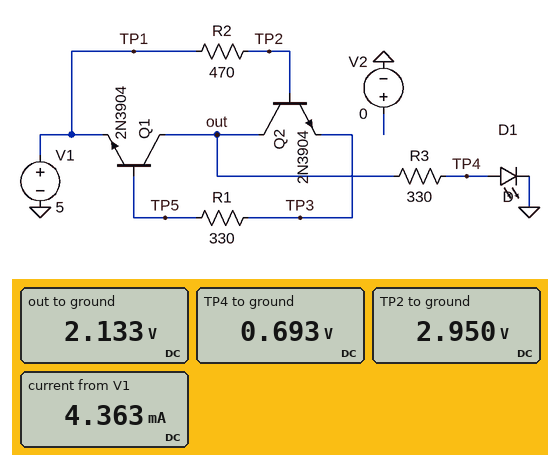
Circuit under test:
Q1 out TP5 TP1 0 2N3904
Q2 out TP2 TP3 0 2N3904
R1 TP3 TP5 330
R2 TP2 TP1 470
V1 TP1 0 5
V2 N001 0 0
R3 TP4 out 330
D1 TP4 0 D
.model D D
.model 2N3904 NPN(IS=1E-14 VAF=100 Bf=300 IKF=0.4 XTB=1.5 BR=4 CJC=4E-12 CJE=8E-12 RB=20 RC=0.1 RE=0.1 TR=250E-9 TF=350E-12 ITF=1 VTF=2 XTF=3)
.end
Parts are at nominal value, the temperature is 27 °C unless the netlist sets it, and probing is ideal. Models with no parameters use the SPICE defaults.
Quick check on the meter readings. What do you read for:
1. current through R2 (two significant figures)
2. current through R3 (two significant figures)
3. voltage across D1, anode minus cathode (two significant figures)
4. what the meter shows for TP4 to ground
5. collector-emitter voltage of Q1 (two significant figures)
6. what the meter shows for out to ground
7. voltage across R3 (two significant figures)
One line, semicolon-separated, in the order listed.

4.4 mA; 4.4 mA; 690 mV; 0.693 V; -2.9 V; 2.133 V; 1.4 V
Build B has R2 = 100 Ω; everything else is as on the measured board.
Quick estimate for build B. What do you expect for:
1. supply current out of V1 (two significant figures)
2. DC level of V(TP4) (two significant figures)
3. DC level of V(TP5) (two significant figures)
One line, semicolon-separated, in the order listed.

7.9 mA; 710 mV; 3.3 V
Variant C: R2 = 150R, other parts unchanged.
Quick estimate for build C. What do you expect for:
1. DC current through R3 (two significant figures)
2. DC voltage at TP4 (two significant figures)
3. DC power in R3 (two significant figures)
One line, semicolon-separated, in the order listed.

7.1 mA; 710 mV; 17 mW
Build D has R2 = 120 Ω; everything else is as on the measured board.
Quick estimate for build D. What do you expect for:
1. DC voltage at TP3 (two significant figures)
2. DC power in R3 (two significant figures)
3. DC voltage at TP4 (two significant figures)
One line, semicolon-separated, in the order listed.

3.2 V; 19 mW; 710 mV
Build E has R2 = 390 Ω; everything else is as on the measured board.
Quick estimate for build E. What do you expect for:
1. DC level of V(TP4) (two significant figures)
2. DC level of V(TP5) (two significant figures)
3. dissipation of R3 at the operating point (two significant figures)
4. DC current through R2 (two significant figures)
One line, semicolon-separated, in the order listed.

700 mV; 2.3 V; 7.7 mW; 4.8 mA
